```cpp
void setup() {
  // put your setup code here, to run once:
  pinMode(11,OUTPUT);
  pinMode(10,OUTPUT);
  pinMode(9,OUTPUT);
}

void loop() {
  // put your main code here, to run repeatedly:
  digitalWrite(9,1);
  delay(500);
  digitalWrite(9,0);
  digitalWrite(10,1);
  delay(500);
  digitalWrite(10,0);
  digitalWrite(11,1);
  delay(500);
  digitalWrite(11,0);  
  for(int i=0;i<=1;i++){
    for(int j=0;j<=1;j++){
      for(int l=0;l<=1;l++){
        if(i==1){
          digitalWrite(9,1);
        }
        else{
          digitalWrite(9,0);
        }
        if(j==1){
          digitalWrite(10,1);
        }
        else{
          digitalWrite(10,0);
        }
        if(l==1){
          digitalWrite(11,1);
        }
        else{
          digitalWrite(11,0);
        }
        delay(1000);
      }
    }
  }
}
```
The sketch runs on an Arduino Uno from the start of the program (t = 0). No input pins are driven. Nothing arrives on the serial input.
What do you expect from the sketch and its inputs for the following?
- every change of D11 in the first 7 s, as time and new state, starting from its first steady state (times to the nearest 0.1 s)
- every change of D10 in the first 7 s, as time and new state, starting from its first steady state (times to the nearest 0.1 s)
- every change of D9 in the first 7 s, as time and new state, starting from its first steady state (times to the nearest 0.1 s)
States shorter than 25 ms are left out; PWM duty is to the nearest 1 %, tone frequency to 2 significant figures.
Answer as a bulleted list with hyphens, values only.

- 0 s low; 1 s high; 1.5 s low; 2.5 s high; 3.5 s low; 4.5 s high; 5.5 s low; 6.5 s high
- 0 s low; 0.5 s high; 1 s low; 3.5 s high; 5.5 s low
- 0 s high; 0.5 s low; 5.5 s high
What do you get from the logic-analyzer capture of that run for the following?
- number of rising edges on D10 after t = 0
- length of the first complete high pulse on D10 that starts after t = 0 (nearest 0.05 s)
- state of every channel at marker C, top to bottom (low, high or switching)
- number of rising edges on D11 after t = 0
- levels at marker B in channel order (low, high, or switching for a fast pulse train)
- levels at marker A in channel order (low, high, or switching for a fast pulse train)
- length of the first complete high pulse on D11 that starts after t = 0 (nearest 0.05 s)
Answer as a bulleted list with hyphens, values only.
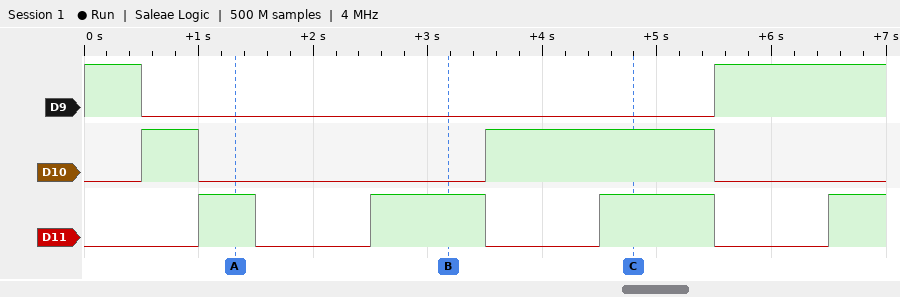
- 2
- 0.50 s
- D9 low, D10 high, D11 high
- 4
- D9 low, D10 low, D11 high
- D9 low, D10 low, D11 high
- 0.50 s
